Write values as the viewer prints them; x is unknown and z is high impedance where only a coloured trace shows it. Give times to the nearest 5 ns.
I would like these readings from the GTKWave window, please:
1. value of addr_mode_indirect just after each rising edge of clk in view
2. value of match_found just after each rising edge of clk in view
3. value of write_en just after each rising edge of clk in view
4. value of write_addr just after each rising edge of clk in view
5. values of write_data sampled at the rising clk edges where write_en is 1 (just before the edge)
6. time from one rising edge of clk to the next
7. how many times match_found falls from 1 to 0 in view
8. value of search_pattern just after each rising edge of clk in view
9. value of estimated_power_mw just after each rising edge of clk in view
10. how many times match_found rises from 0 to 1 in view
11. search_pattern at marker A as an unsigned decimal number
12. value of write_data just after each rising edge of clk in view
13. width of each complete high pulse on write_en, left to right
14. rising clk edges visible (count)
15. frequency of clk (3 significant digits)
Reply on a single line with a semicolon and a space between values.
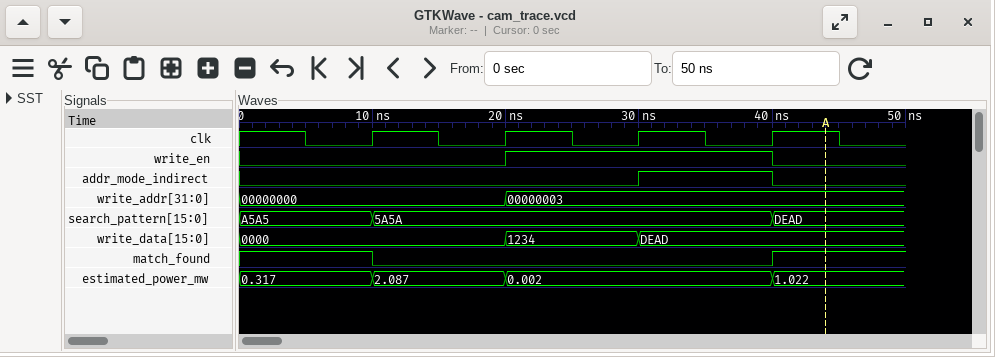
0 0 1 0; 0 0 0 1; 0 1 1 0; 00000000, 00000003, 00000003, 00000003; 1234, DEAD; 10 ns; 1; 5A5A, 5A5A, 5A5A, DEAD; 2.087, 0.002, 0.002, 1.022; 1; 57005; 0000, 1234, DEAD, DEAD; 20 ns; 4; 100 MHz
